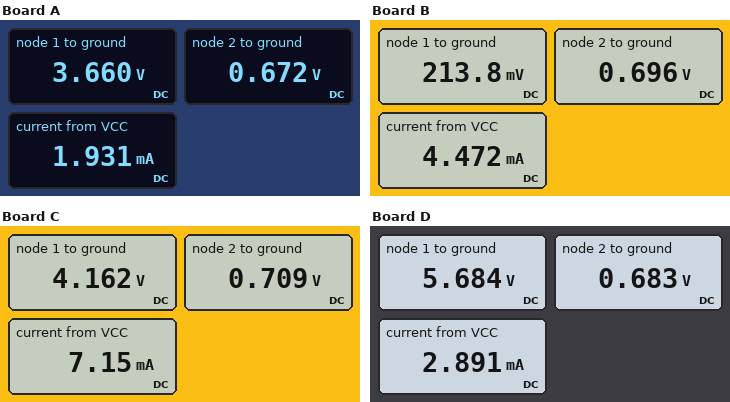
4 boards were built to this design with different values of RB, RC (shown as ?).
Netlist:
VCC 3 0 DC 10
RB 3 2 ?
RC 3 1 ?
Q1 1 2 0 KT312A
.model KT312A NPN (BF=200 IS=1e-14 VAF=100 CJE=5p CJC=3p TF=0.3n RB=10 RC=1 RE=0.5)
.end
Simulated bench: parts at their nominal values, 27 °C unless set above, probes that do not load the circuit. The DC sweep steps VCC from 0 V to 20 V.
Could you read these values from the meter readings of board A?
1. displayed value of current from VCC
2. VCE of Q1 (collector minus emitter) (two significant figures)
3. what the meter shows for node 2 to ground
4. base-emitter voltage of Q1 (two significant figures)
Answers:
1.931 mA
3.7 V
0.672 V
670 mV
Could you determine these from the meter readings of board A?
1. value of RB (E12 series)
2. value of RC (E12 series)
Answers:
1 MΩ
3.3 kΩ
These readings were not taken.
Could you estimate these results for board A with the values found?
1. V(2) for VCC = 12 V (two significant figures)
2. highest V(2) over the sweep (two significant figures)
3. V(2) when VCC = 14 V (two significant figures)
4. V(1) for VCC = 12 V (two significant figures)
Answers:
680 mV
690 mV
680 mV
4.3 V
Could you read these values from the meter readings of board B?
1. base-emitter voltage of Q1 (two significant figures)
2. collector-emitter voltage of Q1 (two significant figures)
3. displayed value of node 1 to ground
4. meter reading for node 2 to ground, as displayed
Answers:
700 mV
210 mV
213.8 mV
0.696 V
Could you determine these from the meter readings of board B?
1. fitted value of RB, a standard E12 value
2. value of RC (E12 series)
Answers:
390 kΩ
2.2 kΩ
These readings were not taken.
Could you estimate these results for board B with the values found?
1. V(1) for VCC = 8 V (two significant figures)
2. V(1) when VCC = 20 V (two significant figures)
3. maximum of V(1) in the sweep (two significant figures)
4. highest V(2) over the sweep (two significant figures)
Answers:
220 mV
210 mV
570 mV
720 mV
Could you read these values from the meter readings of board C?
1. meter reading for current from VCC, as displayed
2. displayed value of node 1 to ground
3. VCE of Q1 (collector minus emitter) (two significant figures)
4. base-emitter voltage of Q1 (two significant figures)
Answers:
7.15 mA
4.162 V
4.2 V
710 mV
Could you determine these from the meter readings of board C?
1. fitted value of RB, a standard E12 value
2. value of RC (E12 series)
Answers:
270 kΩ
820 Ω
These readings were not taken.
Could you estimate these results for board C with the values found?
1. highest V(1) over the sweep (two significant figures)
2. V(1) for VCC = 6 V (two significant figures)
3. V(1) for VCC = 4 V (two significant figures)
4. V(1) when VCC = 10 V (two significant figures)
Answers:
7.5 V
2.7 V
2.0 V
4.2 V
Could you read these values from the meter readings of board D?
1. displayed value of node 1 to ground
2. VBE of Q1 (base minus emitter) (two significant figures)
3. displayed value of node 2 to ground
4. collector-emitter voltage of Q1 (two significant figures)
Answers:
5.684 V
680 mV
0.683 V
5.7 V
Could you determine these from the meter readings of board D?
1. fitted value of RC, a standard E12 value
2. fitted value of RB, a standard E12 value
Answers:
1.5 kΩ
680 kΩ
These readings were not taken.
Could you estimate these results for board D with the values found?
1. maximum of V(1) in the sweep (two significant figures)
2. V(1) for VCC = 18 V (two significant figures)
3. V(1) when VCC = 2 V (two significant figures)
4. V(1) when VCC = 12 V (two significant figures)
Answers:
11 V
9.7 V
1.4 V
6.7 V
